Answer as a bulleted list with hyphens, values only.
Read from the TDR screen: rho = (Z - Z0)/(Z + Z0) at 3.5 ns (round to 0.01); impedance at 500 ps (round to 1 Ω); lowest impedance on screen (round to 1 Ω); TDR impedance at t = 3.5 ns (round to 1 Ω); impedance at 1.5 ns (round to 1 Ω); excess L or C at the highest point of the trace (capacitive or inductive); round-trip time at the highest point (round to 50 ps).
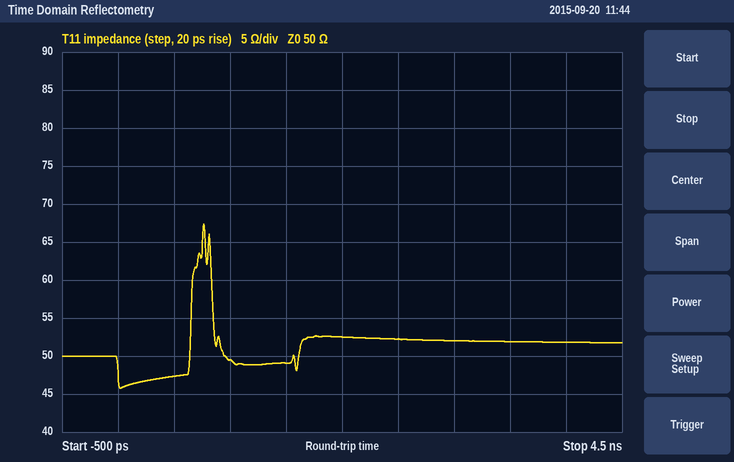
- +0.02
- 47 Ω
- 46 Ω
- 52 Ω
- 49 Ω
- inductive
- 750 ps
